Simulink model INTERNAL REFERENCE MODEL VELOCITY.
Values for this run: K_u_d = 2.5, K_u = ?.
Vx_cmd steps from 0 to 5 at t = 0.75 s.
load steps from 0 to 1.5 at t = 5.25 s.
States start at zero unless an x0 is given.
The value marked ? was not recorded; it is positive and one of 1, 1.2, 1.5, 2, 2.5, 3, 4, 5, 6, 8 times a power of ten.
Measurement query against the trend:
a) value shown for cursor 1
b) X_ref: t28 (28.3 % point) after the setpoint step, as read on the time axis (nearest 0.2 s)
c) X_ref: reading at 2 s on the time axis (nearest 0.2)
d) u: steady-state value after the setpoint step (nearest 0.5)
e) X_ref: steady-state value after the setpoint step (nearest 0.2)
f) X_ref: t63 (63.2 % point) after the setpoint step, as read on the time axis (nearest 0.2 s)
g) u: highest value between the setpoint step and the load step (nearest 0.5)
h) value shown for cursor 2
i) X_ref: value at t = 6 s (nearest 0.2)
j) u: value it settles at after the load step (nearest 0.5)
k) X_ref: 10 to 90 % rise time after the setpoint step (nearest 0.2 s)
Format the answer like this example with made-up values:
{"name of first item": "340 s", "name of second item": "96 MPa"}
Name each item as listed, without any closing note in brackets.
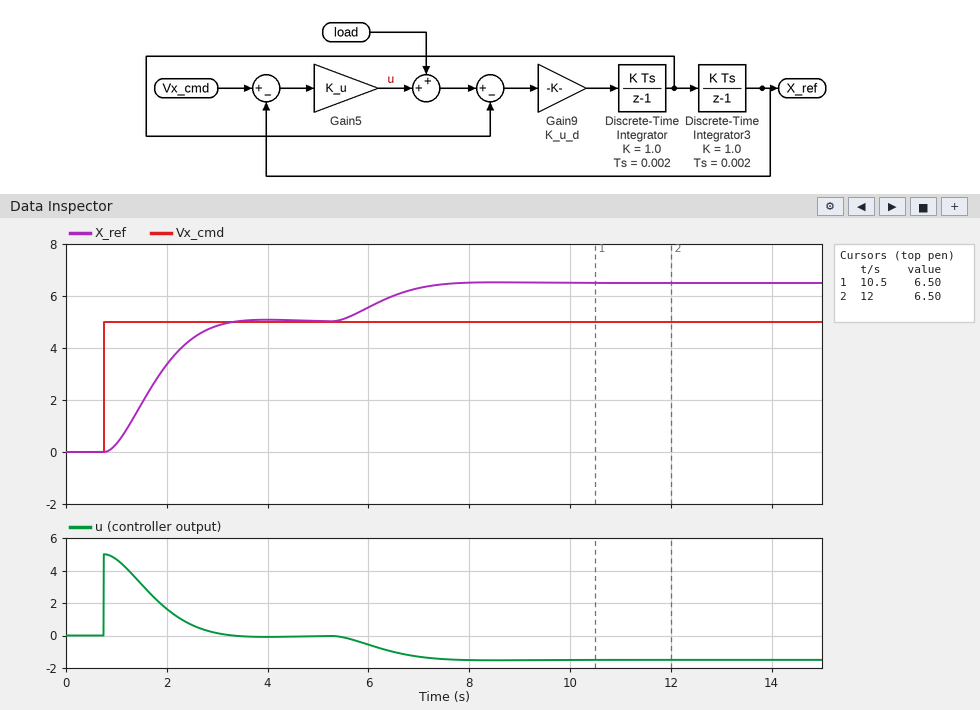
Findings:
{"value shown for cursor 1": "6.50", "X_ref: t28 (28.3 % point) after the setpoint step, as read on the time axis": "1.4 s", "X_ref: reading at 2 s on the time axis": "3.4", "u: steady-state value after the setpoint step": "0.0", "X_ref: steady-state value after the setpoint step": "5.0", "X_ref: t63 (63.2 % point) after the setpoint step, as read on the time axis": "2.0 s", "u: highest value between the setpoint step and the load step": "5.0", "value shown for cursor 2": "6.50", "X_ref: value at t = 6 s": "5.6", "u: value it settles at after the load step": "-1.5", "X_ref: 10 to 90 % rise time after the setpoint step": "1.6 s"}
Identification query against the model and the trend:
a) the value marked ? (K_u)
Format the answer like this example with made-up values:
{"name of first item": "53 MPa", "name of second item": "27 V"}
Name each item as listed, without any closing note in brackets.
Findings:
{"the value marked ?": "1"}
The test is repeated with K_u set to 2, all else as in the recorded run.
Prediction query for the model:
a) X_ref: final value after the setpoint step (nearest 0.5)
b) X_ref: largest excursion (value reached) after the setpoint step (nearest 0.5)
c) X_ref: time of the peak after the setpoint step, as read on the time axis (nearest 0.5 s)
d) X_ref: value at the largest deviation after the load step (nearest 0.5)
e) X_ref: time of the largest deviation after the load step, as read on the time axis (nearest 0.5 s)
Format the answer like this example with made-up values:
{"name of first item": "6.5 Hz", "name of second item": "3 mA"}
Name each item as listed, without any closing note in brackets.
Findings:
{"X_ref: final value after the setpoint step": "5.0", "X_ref: largest excursion (value reached) after the setpoint step": "5.5", "X_ref: time of the peak after the setpoint step, as read on the time axis": "2.5 s", "X_ref: value at the largest deviation after the load step": "6.0", "X_ref: time of the largest deviation after the load step, as read on the time axis": "7.0 s"}
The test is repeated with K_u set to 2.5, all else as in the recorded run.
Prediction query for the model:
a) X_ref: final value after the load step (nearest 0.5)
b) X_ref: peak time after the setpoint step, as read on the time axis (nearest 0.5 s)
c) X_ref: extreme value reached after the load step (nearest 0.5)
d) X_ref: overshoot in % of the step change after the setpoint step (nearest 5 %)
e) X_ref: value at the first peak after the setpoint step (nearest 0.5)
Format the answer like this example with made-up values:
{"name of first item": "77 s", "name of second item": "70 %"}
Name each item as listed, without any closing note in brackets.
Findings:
{"X_ref: final value after the load step": "5.5", "X_ref: peak time after the setpoint step, as read on the time axis": "2.0 s", "X_ref: extreme value reached after the load step": "5.5", "X_ref: overshoot in % of the step change after the setpoint step": "15 %", "X_ref: value at the first peak after the setpoint step": "6.0"}
